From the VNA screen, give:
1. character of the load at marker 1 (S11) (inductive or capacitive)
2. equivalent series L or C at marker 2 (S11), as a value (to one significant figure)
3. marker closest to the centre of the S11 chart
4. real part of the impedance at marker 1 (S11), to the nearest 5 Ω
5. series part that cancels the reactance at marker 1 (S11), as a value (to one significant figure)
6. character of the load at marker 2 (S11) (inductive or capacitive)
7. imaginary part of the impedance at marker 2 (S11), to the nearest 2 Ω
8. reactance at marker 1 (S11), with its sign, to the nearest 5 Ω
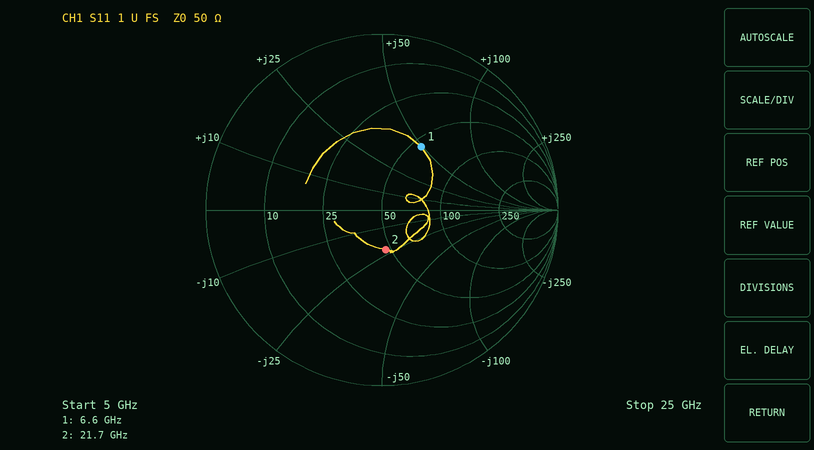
inductive
300 fF
marker 2
55 Ω
500 fF
capacitive
-22 Ω
+50 Ω
